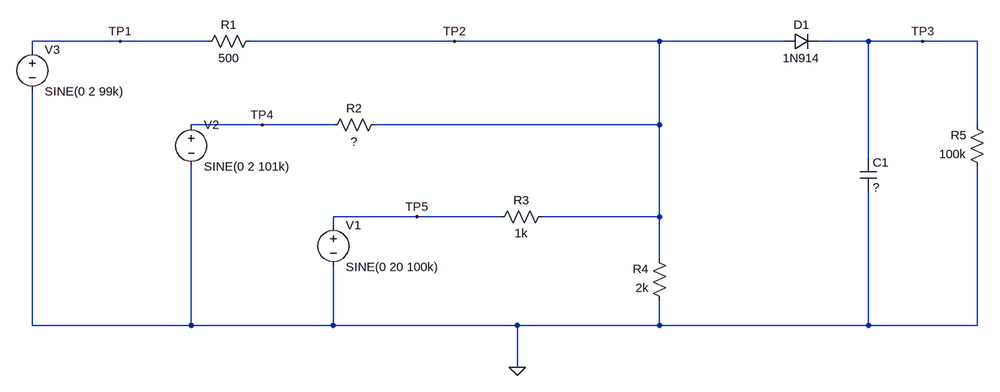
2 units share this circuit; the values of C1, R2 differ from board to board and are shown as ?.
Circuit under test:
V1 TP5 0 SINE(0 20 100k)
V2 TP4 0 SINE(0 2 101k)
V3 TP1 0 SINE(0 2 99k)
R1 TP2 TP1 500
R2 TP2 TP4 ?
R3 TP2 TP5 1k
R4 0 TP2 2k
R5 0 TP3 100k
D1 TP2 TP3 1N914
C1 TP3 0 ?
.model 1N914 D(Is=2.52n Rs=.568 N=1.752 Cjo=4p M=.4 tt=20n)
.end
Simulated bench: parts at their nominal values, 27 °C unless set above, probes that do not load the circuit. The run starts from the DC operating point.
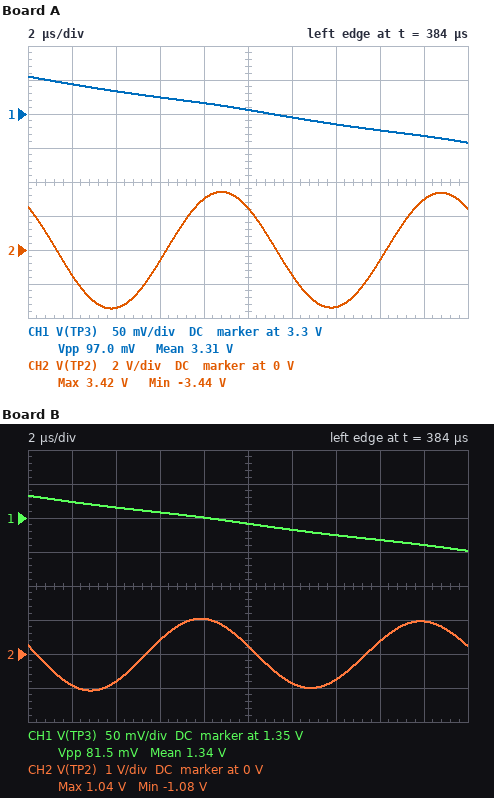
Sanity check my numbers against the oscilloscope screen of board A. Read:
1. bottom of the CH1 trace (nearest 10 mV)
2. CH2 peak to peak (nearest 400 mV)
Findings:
3.26 V
6.8 V
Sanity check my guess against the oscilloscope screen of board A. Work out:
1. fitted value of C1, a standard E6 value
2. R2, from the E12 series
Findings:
6.8 nF
1 kΩ
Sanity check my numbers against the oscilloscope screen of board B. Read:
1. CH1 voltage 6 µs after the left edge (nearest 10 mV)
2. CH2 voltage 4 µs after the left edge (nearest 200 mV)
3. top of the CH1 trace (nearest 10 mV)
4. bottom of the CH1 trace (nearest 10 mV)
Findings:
1.36 V
-800 mV
1.38 V
1.30 V
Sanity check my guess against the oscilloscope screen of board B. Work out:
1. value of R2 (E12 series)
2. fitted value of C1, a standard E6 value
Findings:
180 Ω
3.3 nF
